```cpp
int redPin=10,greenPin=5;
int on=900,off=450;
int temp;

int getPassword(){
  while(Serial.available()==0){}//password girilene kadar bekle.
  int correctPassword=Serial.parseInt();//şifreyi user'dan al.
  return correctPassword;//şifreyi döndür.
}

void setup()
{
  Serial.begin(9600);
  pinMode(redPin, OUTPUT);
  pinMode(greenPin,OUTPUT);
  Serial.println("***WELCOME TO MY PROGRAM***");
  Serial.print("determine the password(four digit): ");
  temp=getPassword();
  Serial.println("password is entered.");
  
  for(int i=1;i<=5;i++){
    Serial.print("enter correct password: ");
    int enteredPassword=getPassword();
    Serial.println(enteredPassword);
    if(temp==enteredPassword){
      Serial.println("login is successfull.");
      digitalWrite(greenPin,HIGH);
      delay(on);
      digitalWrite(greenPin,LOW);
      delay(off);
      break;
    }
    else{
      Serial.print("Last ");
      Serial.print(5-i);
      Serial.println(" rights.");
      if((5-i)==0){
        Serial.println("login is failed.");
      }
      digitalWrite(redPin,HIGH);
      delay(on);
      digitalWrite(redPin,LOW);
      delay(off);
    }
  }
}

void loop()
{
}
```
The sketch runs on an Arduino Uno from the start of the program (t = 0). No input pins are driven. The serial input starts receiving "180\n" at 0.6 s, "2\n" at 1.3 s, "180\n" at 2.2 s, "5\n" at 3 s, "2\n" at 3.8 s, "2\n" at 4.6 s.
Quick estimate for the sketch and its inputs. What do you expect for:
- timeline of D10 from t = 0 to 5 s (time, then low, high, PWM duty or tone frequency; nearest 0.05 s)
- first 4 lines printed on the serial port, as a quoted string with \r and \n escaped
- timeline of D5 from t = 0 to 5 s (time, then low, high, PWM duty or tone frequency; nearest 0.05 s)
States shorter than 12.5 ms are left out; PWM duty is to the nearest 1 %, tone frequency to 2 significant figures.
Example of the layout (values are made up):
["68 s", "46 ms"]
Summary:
["0 s low; 1.3 s high; 2.2 s low", "\"***WELCOME TO MY PROGRAM***\\r\\ndetermine the password(four digit): password is entered.\\r\\nenter correct password: 2\\r\\nLast 4 rights.\\r\\n\"", "0 s low; 2.65 s high; 3.55 s low"]
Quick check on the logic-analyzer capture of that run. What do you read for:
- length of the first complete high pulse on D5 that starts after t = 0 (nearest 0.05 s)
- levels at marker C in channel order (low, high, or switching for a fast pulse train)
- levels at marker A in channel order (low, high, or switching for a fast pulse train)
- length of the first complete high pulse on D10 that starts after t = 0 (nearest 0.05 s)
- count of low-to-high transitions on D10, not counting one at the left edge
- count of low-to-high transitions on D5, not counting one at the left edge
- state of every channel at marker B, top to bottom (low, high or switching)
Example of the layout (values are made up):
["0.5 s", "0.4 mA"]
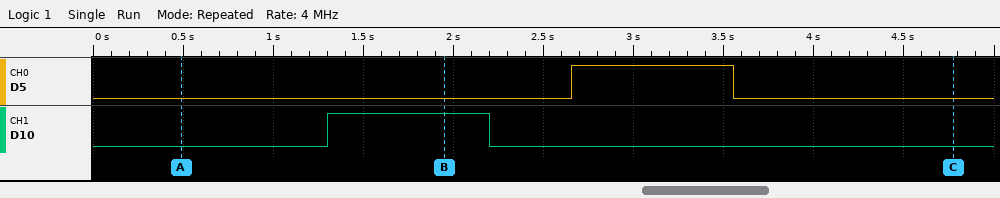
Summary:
["0.90 s", "D5 low, D10 low", "D5 low, D10 low", "0.90 s", "1", "1", "D5 low, D10 high"]
